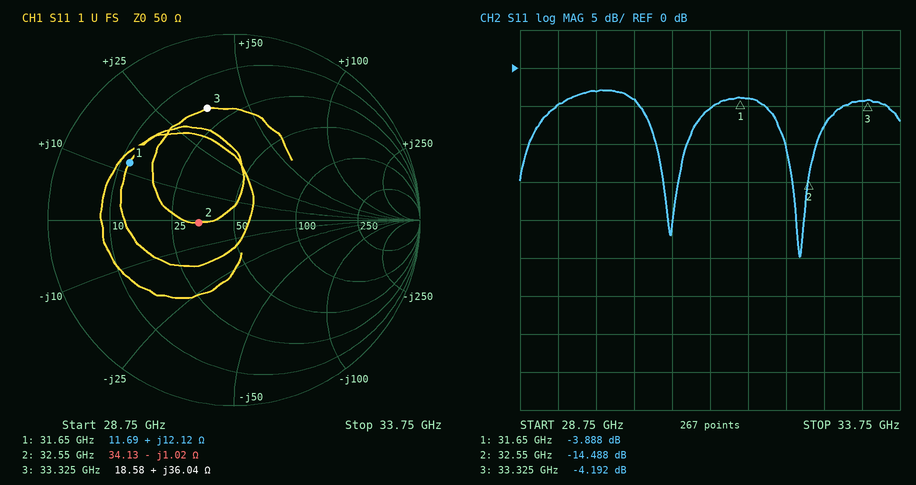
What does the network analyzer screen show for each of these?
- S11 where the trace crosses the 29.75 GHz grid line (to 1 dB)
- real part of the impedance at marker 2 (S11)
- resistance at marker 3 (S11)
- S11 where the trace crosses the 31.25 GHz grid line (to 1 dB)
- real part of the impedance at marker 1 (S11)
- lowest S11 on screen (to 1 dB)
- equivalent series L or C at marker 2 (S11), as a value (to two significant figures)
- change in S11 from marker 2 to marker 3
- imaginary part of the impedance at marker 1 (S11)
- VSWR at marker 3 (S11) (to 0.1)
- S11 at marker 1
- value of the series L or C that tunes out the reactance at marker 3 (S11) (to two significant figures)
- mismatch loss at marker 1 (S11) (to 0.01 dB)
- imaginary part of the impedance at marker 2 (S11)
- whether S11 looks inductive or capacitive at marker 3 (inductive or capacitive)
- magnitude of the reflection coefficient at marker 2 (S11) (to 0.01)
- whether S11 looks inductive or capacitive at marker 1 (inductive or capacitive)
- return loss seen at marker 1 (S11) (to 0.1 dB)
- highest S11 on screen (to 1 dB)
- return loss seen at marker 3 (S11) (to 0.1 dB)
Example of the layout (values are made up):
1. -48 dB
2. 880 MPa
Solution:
1. -3 dB
2. 34.13 Ω
3. 18.58 Ω
4. -5 dB
5. 11.69 Ω
6. -25 dB
7. 4.8 pF
8. 10.296 dB
9. +12.12 Ω
10. 4.2
11. -3.888 dB
12. 130 fF
13. 2.28 dB
14. -1.02 Ω
15. inductive
16. 0.19
17. inductive
18. 3.9 dB
19. -3 dB
20. 4.2 dB
